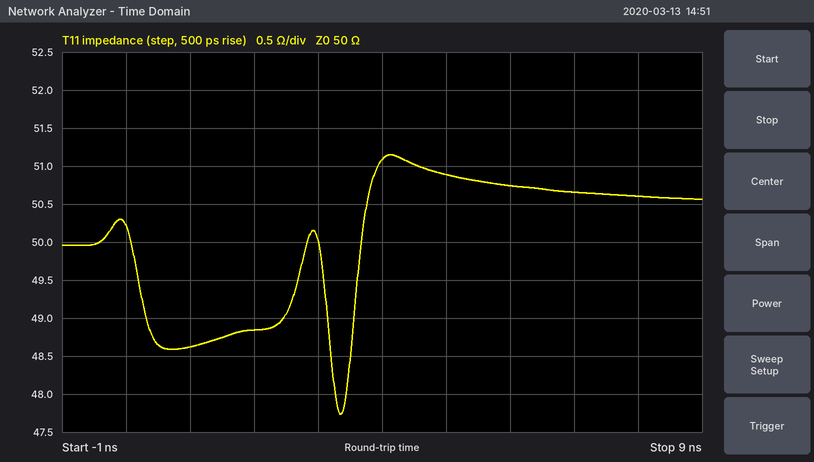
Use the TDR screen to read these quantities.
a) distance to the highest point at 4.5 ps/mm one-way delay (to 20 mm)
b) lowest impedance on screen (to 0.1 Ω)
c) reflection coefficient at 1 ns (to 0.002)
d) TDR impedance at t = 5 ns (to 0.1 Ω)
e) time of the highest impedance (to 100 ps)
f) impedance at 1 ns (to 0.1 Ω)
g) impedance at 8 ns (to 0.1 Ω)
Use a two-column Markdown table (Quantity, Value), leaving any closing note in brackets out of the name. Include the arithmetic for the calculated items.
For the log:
| Quantity | Value |
|---|---|
| distance to the highest point at 4.5 ps/mm one-way delay | 4.1 ns / 2 / 4.5 ps/mm ≈ 456 mm, so 460 mm to the nearest 20 mm |
| lowest impedance on screen | 47.7 Ω |
| reflection coefficient at 1 ns | (48.6 − 50)/(48.6 + 50) ≈ -0.014 |
| TDR impedance at t = 5 ns | 50.9 Ω |
| time of the highest impedance | 4.1 ns |
| impedance at 1 ns | 48.6 Ω |
| impedance at 8 ns | 50.6 Ω |
